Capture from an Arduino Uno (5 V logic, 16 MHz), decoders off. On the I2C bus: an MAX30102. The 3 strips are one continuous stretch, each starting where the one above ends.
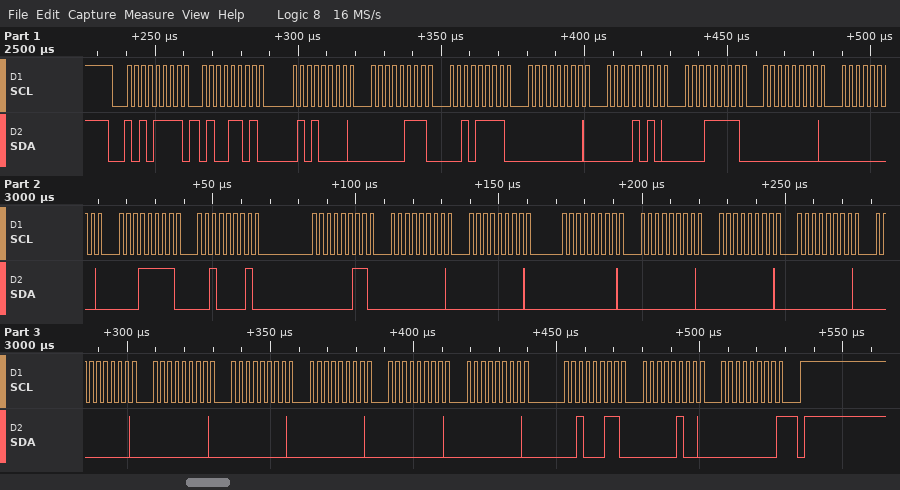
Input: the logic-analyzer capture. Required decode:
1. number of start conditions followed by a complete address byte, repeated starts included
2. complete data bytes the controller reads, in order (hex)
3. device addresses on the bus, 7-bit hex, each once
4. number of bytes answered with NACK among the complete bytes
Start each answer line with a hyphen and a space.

- 1
- 4D 50 07 2F 00 0A 1F 00 00 1F 21 03 00 00 00 00 00 00 00 00 00 00 00 00 23 04 00
- 0x57
- 1
